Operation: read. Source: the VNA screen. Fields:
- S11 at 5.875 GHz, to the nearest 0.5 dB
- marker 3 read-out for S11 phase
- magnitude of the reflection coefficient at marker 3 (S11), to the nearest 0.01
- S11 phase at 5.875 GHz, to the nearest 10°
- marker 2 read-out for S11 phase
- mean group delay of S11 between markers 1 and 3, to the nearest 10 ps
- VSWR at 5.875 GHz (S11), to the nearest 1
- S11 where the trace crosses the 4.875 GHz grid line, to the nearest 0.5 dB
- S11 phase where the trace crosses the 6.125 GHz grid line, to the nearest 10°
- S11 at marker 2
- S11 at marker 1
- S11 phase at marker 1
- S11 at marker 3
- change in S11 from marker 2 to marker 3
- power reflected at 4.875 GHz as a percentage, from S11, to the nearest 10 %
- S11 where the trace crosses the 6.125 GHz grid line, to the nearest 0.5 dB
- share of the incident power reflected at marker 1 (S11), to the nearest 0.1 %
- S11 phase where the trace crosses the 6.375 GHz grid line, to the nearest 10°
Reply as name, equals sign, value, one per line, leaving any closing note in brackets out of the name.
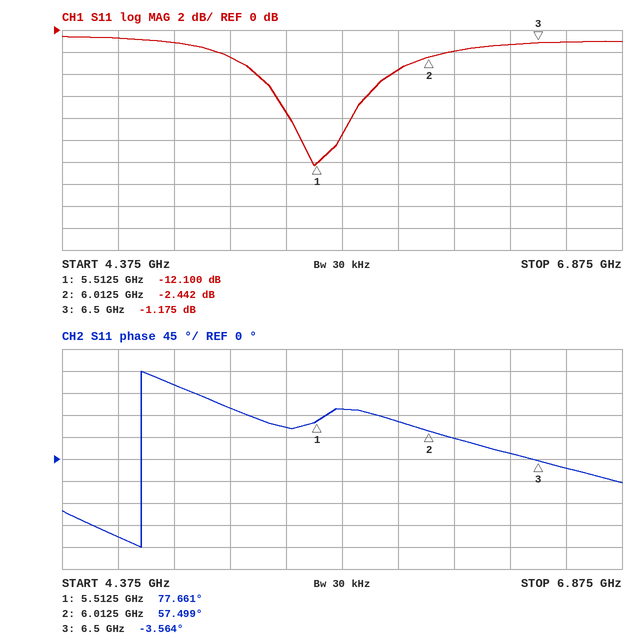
S11 at 5.875 GHz, to the nearest 0.5 dB = -3.5 dB
marker 3 read-out for S11 phase = -3.564°
magnitude of the reflection coefficient at marker 3 (S11), to the nearest 0.01 = 0.87
S11 phase at 5.875 GHz, to the nearest 10° = 80°
marker 2 read-out for S11 phase = 57.499°
mean group delay of S11 between markers 1 and 3, to the nearest 10 ps = 230 ps
VSWR at 5.875 GHz (S11), to the nearest 1 = 5
S11 where the trace crosses the 4.875 GHz grid line, to the nearest 0.5 dB = -1.0 dB
S11 phase where the trace crosses the 6.125 GHz grid line, to the nearest 10° = 40°
S11 at marker 2 = -2.442 dB
S11 at marker 1 = -12.100 dB
S11 phase at marker 1 = 77.661°
S11 at marker 3 = -1.175 dB
change in S11 from marker 2 to marker 3 = 1.267 dB
power reflected at 4.875 GHz as a percentage, from S11, to the nearest 10 % = 80 %
S11 where the trace crosses the 6.125 GHz grid line, to the nearest 0.5 dB = -2.0 dB
share of the incident power reflected at marker 1 (S11), to the nearest 0.1 % = 6.2 %
S11 phase where the trace crosses the 6.375 GHz grid line, to the nearest 10° = 10°
